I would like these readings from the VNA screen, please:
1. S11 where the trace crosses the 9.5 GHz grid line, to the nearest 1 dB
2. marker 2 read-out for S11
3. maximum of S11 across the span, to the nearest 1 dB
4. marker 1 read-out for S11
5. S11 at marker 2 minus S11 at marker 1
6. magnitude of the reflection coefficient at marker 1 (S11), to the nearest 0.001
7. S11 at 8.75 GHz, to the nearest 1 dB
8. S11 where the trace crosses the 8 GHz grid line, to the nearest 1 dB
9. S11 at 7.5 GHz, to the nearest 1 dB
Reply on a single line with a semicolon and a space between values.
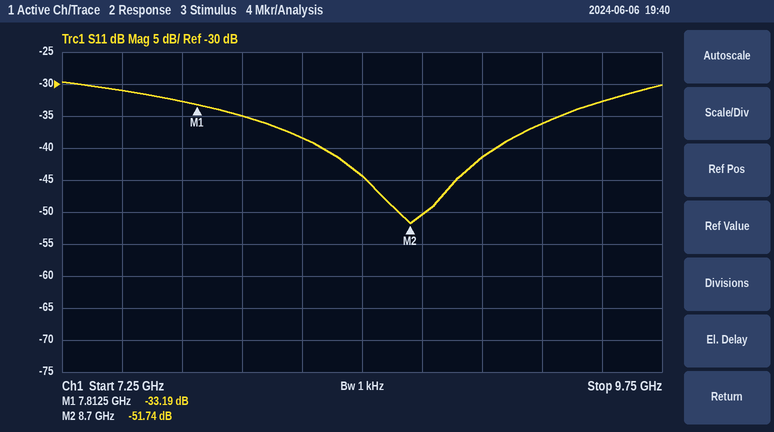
-33 dB; -51.74 dB; -30 dB; -33.19 dB; -18.55 dB; 0.022; -50 dB; -35 dB; -31 dB
